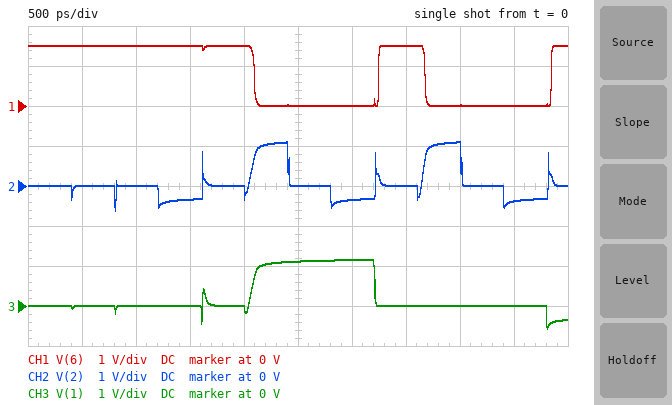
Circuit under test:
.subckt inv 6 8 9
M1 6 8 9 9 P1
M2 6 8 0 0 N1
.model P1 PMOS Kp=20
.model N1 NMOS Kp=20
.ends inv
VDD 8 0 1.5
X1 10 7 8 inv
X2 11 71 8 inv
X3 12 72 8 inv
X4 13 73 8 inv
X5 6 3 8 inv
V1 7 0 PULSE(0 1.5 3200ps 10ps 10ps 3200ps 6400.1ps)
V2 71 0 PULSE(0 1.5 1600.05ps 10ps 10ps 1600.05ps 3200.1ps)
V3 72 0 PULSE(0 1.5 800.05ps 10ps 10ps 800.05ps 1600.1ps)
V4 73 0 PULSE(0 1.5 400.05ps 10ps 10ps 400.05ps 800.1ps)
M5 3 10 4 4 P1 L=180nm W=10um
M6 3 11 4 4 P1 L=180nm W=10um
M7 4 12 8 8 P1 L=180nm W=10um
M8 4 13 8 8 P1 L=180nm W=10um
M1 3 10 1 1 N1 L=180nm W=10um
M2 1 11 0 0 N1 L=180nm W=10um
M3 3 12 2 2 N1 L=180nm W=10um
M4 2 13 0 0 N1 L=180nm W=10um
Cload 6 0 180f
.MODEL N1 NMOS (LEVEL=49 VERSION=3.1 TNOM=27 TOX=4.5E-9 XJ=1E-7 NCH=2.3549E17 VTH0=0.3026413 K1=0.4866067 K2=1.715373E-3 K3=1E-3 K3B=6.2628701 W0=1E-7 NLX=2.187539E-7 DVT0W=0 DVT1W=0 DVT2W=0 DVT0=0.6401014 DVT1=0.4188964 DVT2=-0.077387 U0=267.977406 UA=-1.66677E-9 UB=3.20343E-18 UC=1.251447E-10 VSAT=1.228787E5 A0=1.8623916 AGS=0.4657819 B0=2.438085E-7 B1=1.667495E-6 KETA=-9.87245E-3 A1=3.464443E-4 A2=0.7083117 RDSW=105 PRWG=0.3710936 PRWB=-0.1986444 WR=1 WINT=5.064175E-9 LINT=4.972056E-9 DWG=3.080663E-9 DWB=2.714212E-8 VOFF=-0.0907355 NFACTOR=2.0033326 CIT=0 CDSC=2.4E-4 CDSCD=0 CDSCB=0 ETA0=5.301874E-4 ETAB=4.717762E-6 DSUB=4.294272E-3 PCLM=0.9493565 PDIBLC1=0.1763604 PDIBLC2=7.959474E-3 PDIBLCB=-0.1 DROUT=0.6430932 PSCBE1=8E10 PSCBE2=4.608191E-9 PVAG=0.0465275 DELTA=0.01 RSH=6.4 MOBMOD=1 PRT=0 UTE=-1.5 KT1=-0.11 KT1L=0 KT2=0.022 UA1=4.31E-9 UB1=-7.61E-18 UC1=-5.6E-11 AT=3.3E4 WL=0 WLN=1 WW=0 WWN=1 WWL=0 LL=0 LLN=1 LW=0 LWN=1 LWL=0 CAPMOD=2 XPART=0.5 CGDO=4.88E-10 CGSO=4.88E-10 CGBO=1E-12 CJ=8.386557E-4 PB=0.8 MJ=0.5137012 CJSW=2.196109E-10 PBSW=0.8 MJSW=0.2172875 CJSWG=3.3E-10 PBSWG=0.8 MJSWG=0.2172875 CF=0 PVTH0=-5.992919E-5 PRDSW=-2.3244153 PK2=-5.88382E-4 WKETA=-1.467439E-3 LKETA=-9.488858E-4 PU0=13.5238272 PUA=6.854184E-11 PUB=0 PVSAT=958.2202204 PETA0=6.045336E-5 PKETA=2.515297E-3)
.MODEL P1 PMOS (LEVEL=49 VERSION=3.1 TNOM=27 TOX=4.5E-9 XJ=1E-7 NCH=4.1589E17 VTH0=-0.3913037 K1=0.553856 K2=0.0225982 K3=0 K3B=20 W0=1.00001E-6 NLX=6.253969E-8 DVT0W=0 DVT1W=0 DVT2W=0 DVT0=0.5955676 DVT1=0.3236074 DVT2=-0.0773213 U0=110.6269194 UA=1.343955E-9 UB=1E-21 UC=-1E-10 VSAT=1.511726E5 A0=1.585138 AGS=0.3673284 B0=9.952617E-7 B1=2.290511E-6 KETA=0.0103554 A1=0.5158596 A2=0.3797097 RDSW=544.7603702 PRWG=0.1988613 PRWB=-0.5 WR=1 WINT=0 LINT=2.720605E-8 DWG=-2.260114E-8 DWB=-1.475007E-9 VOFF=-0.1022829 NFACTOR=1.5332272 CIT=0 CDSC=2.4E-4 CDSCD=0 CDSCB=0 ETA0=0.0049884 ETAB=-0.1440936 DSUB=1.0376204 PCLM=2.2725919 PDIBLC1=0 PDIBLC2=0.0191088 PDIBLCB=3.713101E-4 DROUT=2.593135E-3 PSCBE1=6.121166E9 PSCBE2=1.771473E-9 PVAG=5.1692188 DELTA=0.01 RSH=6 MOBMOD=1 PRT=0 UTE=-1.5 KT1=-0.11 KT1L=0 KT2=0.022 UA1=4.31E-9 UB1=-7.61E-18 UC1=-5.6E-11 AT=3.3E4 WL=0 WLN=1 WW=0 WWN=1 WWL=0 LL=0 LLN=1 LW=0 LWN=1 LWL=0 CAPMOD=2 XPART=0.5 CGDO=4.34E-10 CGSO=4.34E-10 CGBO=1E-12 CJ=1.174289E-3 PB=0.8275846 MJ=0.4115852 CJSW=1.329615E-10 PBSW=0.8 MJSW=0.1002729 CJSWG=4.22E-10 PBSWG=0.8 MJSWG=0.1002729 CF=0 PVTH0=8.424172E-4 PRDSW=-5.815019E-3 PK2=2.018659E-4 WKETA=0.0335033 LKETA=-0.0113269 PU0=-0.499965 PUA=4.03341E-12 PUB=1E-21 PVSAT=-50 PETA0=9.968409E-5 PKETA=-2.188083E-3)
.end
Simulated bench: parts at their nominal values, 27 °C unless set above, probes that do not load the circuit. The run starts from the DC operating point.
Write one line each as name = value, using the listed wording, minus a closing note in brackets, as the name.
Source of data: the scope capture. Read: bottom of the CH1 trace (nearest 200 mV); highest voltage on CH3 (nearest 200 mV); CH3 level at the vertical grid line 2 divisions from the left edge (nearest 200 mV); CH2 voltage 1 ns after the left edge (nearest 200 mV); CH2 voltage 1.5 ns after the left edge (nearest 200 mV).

bottom of the CH1 trace = 0 V
highest voltage on CH3 = 1.2 V
CH3 level at the vertical grid line 2 divisions from the left edge = 0 V
CH2 voltage 1 ns after the left edge = 0 V
CH2 voltage 1.5 ns after the left edge = -400 mV
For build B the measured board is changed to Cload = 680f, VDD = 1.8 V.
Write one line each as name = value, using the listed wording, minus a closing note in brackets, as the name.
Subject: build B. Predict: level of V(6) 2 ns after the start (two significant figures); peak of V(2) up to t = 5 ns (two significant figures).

level of V(6) 2 ns after the start = 1.8 V
peak of V(2) up to t = 5 ns = 1.4 V
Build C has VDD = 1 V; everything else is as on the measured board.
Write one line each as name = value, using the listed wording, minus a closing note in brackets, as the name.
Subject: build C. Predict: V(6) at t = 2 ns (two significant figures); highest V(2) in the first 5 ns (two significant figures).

V(6) at t = 2 ns = 1.0 V
highest V(2) in the first 5 ns = 590 mV
